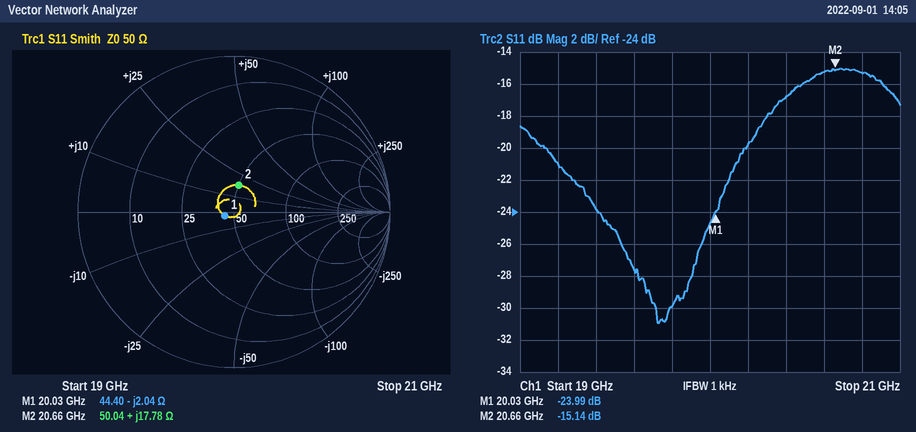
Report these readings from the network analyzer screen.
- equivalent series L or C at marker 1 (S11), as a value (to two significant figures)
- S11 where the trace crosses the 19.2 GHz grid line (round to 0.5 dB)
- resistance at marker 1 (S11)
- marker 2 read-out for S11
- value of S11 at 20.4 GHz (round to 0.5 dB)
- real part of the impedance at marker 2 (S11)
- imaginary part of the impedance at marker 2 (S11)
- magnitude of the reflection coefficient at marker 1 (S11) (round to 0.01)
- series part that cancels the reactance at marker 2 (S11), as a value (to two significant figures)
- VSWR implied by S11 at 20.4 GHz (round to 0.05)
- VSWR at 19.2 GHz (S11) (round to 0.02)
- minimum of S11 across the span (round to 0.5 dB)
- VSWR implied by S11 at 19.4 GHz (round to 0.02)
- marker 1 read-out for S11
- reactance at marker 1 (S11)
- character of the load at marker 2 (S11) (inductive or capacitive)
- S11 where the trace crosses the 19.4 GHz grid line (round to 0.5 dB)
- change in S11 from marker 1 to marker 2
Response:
3.9 pF
-21.0 dB
44.40 Ω
-15.14 dB
-17.0 dB
50.04 Ω
+17.78 Ω
0.06
430 fF
1.35
1.20
-31.0 dB
1.14
-23.99 dB
-2.04 Ω
inductive
-24.0 dB
8.85 dB
